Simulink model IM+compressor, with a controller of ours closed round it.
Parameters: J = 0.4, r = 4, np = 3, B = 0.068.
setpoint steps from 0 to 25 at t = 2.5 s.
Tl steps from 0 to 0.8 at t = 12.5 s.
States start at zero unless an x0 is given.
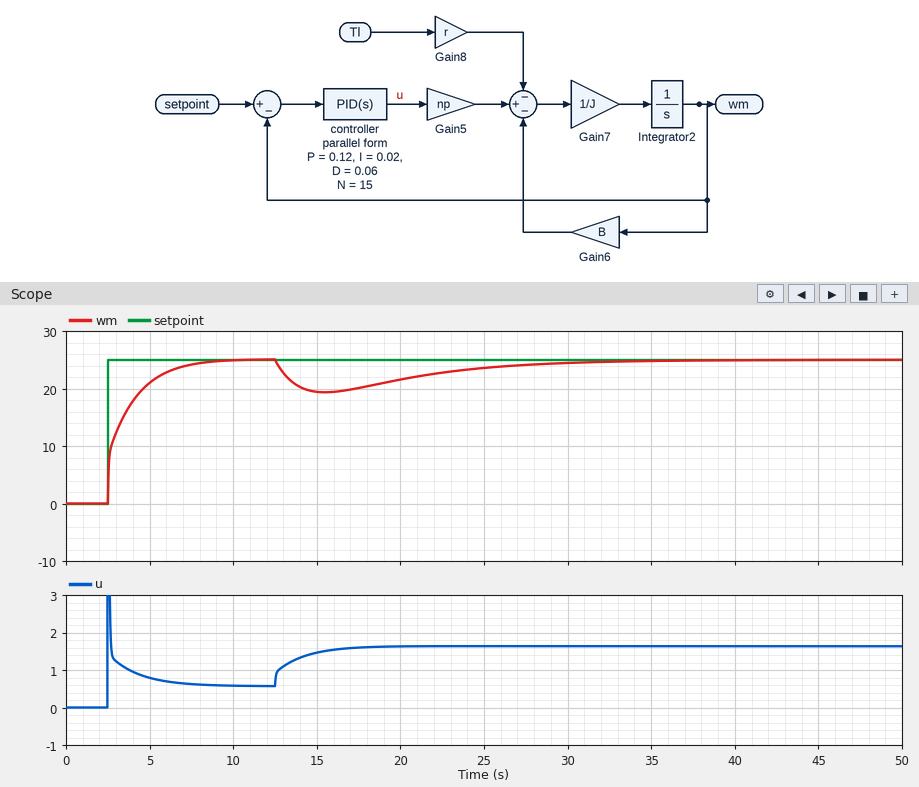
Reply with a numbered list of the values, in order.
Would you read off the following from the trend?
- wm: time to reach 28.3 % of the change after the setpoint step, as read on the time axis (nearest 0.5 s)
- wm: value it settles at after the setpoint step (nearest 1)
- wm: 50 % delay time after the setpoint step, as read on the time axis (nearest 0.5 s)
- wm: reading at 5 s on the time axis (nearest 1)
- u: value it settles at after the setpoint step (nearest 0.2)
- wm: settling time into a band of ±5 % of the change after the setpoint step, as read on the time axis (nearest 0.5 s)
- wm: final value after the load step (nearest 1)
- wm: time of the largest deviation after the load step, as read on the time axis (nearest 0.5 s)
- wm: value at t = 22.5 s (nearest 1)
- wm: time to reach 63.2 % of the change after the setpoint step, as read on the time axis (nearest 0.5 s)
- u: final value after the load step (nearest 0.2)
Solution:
1. 2.5 s
2. 25
3. 3.0 s
4. 21
5. 0.6
6. 7.0 s
7. 25
8. 15.5 s
9. 23
10. 3.5 s
11. 1.6
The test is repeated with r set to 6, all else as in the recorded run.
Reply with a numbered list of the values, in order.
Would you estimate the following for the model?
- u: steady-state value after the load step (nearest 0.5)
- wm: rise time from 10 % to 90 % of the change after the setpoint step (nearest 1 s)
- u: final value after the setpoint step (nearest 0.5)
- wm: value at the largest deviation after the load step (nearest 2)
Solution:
1. 2.0
2. 3 s
3. 0.5
4. 16
